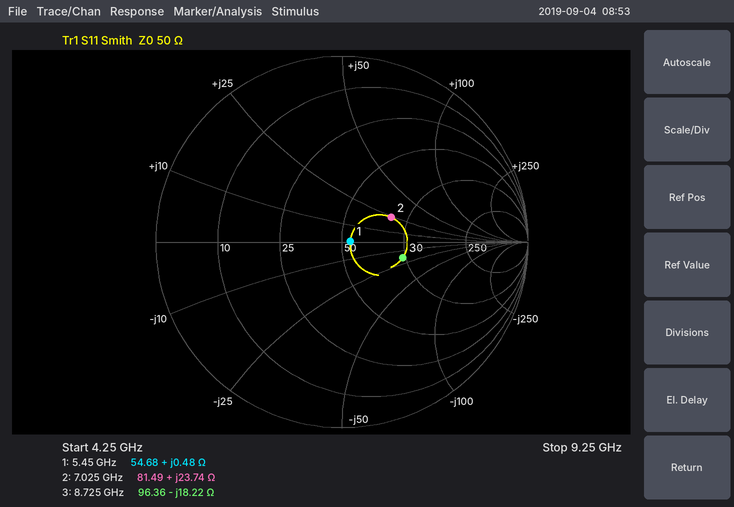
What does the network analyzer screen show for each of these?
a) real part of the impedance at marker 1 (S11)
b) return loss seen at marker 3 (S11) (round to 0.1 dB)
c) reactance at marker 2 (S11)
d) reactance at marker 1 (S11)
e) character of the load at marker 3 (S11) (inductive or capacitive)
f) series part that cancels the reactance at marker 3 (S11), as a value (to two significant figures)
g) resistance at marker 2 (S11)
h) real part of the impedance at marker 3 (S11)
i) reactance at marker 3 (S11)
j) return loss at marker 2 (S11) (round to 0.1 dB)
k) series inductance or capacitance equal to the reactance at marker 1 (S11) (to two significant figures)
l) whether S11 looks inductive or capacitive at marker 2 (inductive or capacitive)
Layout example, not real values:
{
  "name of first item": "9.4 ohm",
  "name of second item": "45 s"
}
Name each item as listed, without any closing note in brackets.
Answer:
{
  "real part of the impedance at marker 1": "54.68 Ω",
  "return loss seen at marker 3 (S11)": "9.4 dB",
  "reactance at marker 2": "+23.74 Ω",
  "reactance at marker 1": "+0.48 Ω",
  "character of the load at marker 3 (S11)": "capacitive",
  "series part that cancels the reactance at marker 3 (S11), as a value": "330 pH",
  "resistance at marker 2": "81.49 Ω",
  "real part of the impedance at marker 3": "96.36 Ω",
  "reactance at marker 3": "-18.22 Ω",
  "return loss at marker 2 (S11)": "10.6 dB",
  "series inductance or capacitance equal to the reactance at marker 1 (S11)": "14 pH",
  "whether S11 looks inductive or capacitive at marker 2": "inductive"
}
